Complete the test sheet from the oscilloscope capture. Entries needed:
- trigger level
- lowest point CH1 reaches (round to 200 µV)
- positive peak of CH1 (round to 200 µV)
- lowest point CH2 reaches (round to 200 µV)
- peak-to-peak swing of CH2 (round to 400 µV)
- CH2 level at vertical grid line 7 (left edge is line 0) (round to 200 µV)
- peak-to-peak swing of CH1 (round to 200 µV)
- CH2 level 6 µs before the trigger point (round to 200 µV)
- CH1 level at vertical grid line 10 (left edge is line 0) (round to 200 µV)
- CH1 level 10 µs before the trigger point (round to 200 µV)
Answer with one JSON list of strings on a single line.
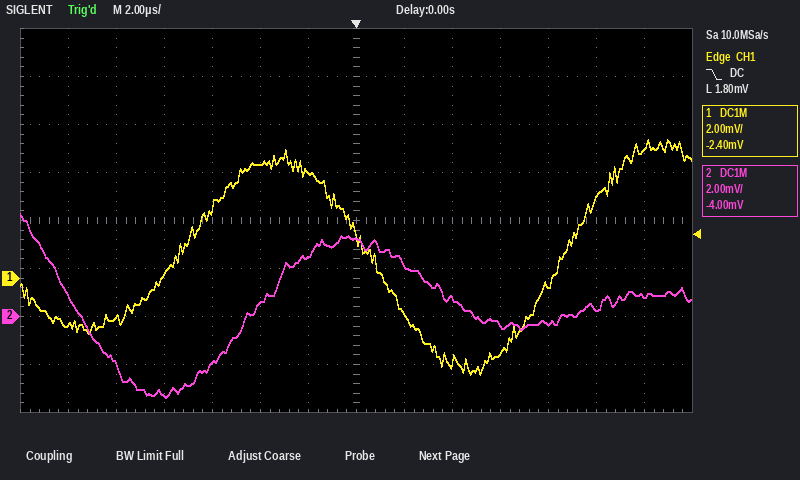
["1.80 mV", "-4.0 mV", "5.8 mV", "-3.4 mV", "7.6 mV", "3.2 mV", "9.8 mV", "-2.0 mV", "-3.2 mV", "-1.6 mV"]
